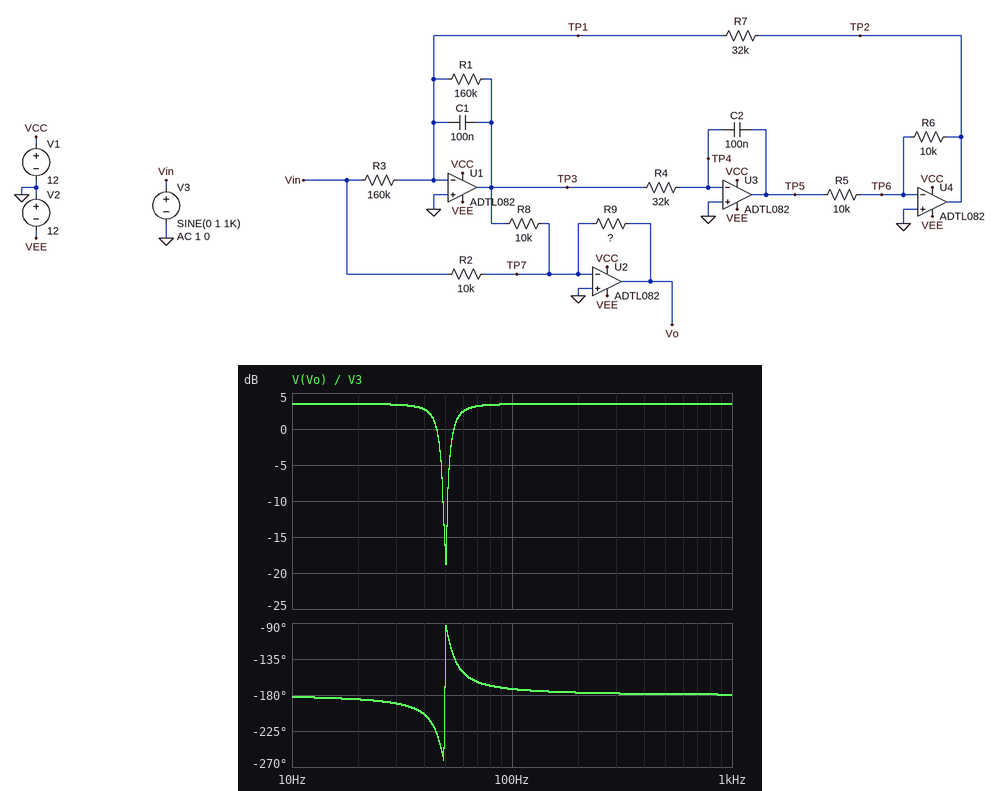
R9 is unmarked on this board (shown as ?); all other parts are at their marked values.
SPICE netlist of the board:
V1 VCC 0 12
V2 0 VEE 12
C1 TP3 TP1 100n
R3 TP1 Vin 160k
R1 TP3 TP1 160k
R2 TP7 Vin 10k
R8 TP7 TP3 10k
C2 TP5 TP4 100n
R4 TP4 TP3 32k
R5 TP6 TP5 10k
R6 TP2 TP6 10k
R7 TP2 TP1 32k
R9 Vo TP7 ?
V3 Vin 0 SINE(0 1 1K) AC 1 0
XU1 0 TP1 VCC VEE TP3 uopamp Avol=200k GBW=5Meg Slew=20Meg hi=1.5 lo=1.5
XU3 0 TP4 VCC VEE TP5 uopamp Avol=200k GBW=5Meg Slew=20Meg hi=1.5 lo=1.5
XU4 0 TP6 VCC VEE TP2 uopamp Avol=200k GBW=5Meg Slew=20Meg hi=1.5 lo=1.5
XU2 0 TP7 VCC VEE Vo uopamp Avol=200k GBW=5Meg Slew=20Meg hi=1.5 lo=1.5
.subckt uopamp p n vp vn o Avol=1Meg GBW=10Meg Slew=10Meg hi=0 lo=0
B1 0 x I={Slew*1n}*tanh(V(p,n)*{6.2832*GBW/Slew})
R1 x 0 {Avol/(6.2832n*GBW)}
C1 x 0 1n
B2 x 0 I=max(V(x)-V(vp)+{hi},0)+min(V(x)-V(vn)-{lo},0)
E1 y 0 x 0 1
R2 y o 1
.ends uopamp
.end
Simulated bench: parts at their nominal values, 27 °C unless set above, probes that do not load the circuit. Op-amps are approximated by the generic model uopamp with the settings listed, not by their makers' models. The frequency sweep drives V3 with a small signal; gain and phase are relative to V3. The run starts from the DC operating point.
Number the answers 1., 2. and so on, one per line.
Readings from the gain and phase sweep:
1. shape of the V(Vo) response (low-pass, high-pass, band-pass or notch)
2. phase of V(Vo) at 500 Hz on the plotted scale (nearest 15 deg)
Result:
1. notch
2. -180 deg
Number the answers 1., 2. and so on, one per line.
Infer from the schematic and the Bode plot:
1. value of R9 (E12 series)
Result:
1. 15 kΩ
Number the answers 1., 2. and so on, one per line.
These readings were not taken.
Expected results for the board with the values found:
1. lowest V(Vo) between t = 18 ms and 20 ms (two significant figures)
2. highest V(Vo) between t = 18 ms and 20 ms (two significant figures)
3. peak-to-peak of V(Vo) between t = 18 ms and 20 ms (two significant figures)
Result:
1. -1.5 V
2. 1.5 V
3. 3.0 V
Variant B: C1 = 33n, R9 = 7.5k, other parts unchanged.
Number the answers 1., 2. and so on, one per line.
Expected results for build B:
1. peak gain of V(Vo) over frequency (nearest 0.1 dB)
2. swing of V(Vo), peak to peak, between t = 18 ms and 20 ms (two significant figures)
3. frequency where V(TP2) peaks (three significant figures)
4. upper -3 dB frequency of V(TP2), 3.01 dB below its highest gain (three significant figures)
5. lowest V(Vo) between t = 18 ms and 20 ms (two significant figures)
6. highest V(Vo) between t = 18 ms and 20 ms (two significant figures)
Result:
1. -2.5 dB
2. 1.5 V
3. 83.9 Hz
4. 98.0 Hz
5. -750 mV
6. 750 mV
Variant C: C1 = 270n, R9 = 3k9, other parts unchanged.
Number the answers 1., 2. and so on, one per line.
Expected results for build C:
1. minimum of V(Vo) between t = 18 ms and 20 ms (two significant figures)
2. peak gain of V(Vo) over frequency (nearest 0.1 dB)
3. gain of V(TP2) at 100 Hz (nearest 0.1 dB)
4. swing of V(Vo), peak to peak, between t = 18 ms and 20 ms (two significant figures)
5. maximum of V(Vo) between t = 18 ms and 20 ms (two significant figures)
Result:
1. -390 mV
2. -8.2 dB
3. -33.9 dB
4. 780 mV
5. 390 mV
